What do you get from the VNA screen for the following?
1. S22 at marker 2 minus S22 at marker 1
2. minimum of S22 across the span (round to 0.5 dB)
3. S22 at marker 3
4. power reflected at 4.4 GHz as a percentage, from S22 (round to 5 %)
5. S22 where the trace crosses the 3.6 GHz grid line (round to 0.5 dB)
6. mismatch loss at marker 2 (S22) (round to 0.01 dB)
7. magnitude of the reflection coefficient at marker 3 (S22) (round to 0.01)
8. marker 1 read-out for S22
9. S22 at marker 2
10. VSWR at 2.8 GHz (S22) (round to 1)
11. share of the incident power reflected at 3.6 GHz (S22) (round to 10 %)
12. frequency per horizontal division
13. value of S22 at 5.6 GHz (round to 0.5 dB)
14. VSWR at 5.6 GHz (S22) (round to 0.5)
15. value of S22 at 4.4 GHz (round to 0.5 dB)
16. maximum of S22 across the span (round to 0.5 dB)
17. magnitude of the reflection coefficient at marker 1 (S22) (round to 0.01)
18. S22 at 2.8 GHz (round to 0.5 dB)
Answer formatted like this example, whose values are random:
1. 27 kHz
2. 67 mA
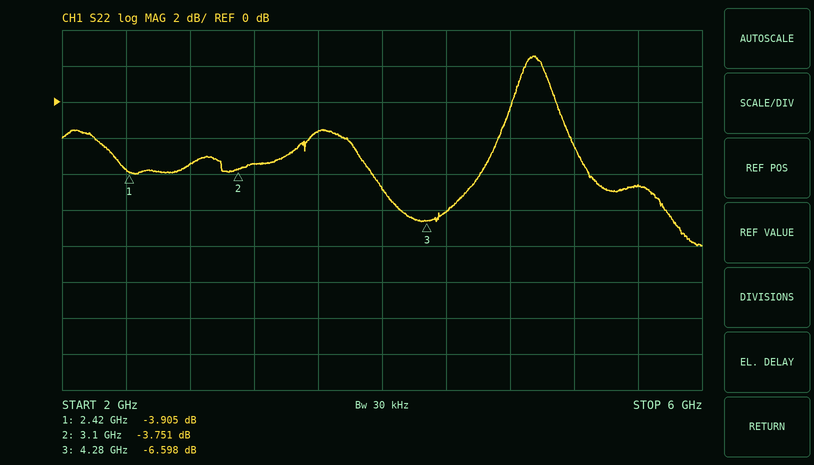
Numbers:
1. 0.154 dB
2. -8.0 dB
3. -6.598 dB
4. 25 %
5. -1.5 dB
6. 2.38 dB
7. 0.47
8. -3.905 dB
9. -3.751 dB
10. 5
11. 70 %
12. 400 MHz
13. -4.5 dB
14. 4.0
15. -6.0 dB
16. 2.5 dB
17. 0.64
18. -3.5 dB
